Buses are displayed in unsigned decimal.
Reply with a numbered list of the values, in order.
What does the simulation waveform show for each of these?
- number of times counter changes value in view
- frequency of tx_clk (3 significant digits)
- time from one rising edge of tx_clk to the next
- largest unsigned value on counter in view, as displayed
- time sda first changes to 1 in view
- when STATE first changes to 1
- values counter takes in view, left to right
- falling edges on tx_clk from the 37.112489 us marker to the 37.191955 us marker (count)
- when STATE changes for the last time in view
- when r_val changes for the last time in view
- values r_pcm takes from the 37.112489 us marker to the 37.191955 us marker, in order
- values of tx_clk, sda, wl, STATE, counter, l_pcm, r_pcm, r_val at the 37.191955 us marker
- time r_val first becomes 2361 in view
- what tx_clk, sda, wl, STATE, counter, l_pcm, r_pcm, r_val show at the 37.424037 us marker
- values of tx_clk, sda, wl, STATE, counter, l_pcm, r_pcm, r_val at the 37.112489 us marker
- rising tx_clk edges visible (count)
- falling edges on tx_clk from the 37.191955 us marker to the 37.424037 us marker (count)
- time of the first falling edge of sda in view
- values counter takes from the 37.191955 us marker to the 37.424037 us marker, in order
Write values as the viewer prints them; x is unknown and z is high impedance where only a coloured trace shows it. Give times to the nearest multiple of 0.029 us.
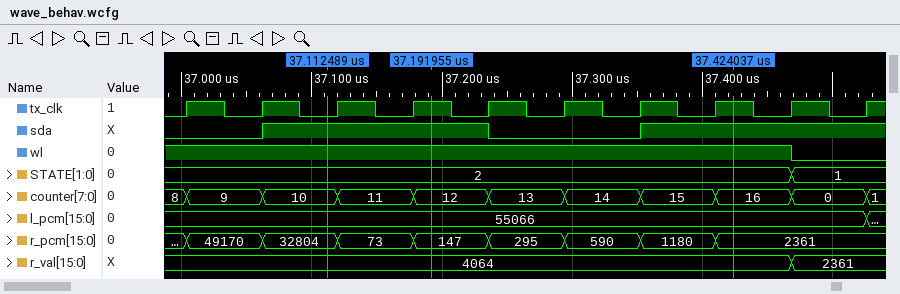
1. 10
2. 17.2 MHz
3. 0.058 us
4. 16
5. 37.062 us
6. 37.468 us
7. 8, 9, 10, 11, 12, 13, 14, 15, 16, 0, 1
8. 1
9. 37.468 us
10. 37.468 us
11. 32804, 73, 147
12. tx_clk=1, sda=1, wl=1, STATE=2, counter=12, l_pcm=55066, r_pcm=147, r_val=4064
13. 37.468 us
14. tx_clk=1, sda=1, wl=1, STATE=2, counter=16, l_pcm=55066, r_pcm=2361, r_val=4064
15. tx_clk=0, sda=1, wl=1, STATE=2, counter=10, l_pcm=55066, r_pcm=32804, r_val=4064
16. 10
17. 4
18. 37.236 us
19. 12, 13, 14, 15, 16
